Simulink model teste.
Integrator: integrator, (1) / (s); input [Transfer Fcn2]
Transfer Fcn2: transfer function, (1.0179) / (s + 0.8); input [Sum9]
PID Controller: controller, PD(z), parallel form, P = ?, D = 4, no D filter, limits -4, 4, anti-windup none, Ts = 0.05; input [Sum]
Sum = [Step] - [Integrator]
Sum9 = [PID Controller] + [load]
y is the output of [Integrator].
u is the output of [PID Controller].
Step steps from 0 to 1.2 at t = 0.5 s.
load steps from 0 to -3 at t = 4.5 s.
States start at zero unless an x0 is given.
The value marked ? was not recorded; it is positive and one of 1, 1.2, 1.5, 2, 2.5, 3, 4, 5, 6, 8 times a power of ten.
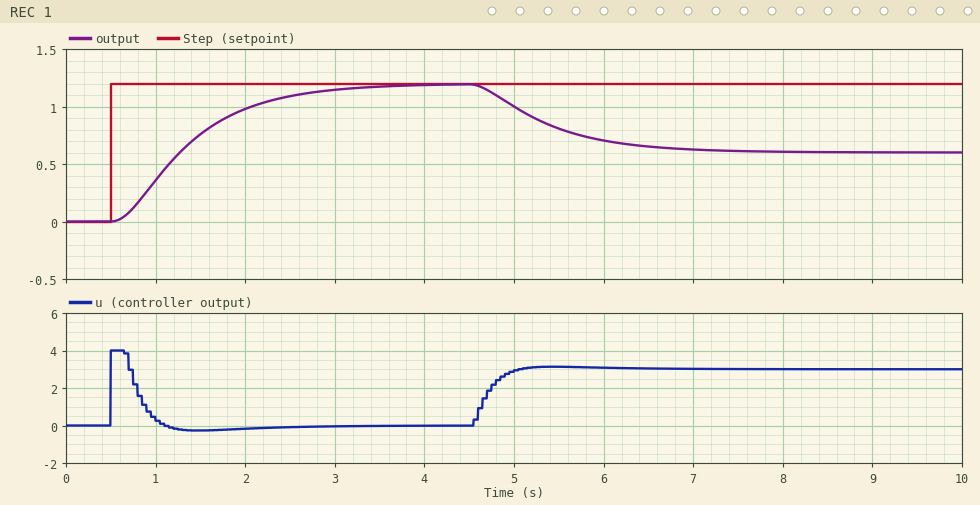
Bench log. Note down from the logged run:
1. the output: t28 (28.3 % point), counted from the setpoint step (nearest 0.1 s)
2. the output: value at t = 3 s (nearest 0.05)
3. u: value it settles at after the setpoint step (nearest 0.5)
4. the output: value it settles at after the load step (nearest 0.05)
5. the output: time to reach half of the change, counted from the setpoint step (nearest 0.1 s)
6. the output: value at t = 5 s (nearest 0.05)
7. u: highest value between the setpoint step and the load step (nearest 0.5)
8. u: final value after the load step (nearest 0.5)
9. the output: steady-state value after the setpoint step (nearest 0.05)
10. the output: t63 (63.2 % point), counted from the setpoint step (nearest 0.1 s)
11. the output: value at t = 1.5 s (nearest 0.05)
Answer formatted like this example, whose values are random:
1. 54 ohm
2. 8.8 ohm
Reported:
1. 0.5 s
2. 1.15
3. 0.0
4. 0.60
5. 0.8 s
6. 1.00
7. 4.0
8. 3.0
9. 1.20
10. 1.0 s
11. 0.75
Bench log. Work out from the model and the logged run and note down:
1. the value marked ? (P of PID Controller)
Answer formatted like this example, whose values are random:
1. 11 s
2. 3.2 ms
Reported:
1. 5
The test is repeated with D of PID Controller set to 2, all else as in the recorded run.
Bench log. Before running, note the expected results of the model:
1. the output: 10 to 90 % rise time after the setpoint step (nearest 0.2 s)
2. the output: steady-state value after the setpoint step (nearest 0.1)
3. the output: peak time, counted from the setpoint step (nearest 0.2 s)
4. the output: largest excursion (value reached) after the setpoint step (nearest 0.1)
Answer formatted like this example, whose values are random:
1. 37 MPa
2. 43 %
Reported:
1. 0.8 s
2. 1.2
3. 1.8 s
4. 1.3
